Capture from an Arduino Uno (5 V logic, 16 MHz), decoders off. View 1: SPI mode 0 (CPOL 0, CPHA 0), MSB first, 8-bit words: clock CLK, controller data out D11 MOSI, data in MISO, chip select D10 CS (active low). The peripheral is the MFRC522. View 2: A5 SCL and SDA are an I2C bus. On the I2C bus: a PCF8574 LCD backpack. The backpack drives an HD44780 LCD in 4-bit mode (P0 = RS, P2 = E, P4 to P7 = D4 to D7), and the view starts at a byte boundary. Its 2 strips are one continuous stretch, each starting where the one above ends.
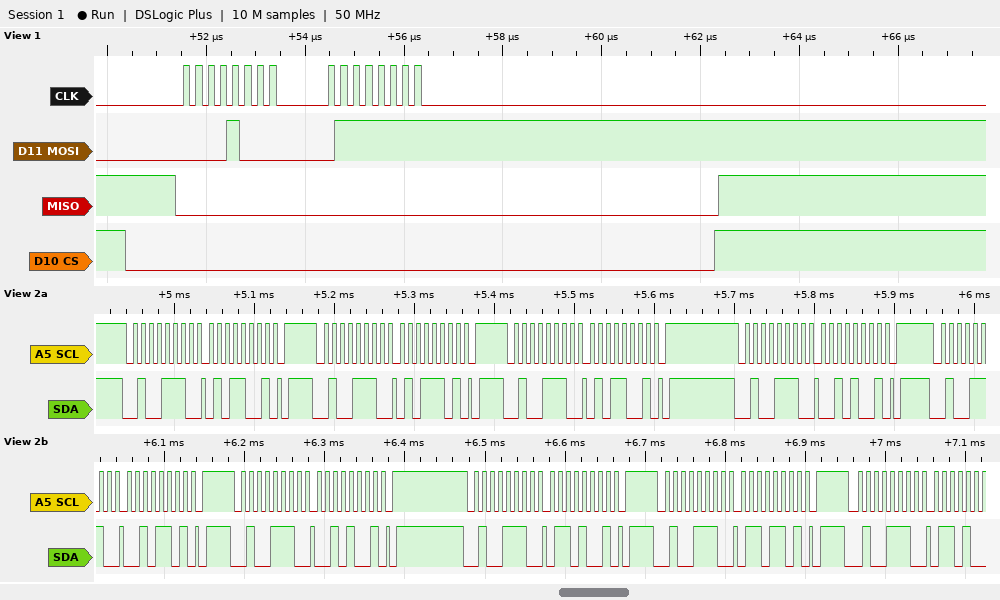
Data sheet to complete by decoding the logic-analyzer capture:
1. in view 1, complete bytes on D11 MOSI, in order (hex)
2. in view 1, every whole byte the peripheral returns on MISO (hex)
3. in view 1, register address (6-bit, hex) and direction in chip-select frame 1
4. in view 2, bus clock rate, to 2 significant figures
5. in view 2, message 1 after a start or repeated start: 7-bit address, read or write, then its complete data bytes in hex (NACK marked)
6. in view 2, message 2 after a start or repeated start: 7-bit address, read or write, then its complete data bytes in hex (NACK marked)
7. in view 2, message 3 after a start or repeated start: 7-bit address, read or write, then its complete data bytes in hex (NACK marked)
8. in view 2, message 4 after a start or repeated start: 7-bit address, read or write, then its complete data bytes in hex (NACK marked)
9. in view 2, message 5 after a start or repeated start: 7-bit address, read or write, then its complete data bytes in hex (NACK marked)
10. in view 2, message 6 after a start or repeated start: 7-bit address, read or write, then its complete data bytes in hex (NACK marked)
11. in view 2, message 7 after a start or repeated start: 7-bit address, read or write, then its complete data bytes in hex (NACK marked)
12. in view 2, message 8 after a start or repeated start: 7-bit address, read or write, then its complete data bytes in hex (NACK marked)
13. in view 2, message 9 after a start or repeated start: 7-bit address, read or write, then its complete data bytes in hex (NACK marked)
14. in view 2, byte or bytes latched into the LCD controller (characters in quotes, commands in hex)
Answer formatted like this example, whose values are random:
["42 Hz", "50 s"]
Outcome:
["08 7F", "00 00", "0x04 write", "100 kHz", "0x27 write: 59", "0x27 write: 5D", "0x27 write: 59", "0x27 write: 29", "0x27 write: 2D", "0x27 write: 29", "0x27 write: 69", "0x27 write: 6D", "0x27 write", "'R'"]
